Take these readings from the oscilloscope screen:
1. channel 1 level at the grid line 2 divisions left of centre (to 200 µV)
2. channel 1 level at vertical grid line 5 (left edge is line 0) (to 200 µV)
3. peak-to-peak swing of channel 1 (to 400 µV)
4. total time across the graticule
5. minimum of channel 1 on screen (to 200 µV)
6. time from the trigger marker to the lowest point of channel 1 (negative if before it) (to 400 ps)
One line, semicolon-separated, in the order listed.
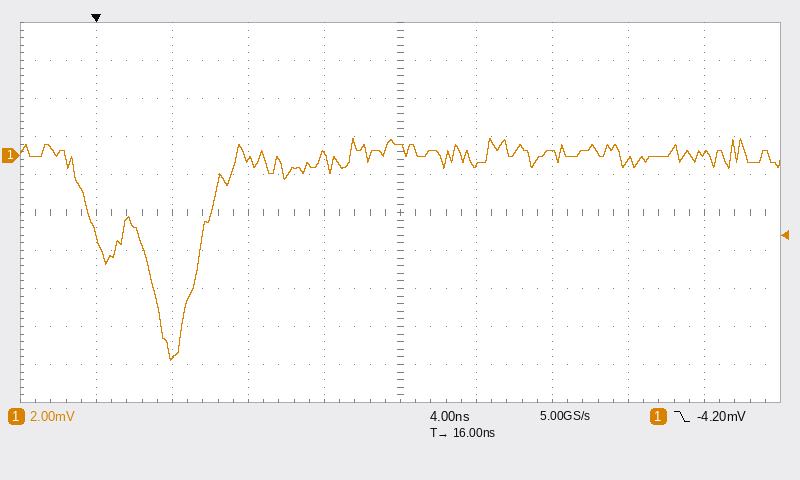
-200 µV; 400 µV; 11.6 mV; 40 ns; -10.8 mV; +4.0 ns
